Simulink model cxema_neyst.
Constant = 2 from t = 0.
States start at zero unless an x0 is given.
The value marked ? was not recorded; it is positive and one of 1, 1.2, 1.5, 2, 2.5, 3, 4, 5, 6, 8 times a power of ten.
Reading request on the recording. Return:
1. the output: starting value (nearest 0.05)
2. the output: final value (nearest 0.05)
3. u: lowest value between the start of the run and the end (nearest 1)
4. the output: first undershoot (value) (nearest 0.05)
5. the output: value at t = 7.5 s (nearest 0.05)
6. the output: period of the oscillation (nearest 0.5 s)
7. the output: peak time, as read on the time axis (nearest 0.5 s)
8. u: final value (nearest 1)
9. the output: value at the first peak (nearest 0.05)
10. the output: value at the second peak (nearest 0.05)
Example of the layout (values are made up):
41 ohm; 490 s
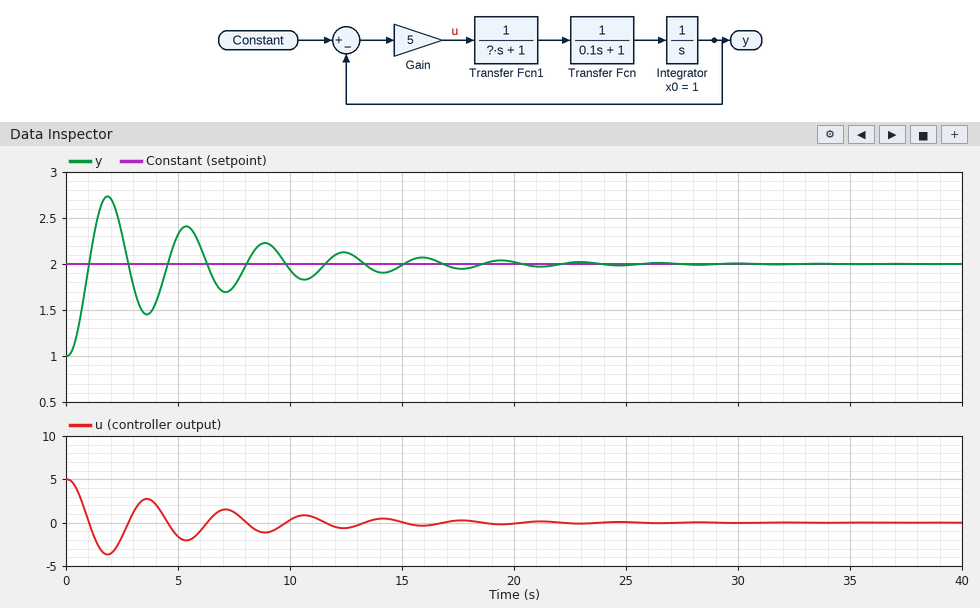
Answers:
1.00; 2.00; -4; 1.45; 1.75; 3.5 s; 2.0 s; 0; 2.75; 2.40
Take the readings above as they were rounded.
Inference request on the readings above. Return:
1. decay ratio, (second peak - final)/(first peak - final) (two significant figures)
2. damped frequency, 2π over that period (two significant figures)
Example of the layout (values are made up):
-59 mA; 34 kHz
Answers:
0.53; 1.8 rad/s
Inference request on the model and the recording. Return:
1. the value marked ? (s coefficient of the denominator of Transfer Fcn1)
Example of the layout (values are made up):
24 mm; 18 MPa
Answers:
1.5
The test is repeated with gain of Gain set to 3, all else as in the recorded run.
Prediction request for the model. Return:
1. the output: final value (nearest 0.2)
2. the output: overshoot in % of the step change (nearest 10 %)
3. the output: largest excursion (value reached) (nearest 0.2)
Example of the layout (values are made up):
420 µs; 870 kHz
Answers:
2.0; 60 %; 2.6
